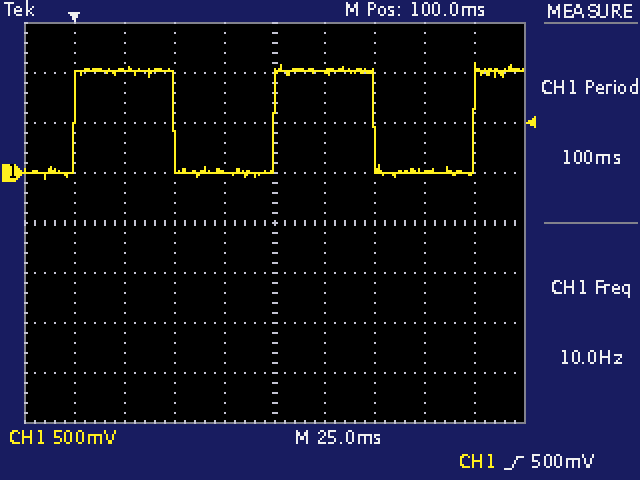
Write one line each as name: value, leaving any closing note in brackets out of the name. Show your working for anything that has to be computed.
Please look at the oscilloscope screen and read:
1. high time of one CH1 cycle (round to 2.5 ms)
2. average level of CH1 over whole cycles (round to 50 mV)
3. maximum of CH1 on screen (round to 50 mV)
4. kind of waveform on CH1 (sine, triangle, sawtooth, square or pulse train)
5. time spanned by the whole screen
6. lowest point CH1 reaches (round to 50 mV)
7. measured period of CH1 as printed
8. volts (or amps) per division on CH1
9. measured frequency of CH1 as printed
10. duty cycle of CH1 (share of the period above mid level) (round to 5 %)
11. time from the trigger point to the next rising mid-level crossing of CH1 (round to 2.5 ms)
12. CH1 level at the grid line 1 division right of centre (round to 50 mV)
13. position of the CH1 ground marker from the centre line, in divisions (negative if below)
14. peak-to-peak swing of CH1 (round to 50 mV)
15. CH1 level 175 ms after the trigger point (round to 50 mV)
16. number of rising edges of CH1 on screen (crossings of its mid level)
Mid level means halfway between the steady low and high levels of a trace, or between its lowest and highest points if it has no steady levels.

high time of one CH1 cycle: 50.0 ms
average level of CH1 over whole cycles: -50 mV + 0.5 × (1.10 V − (-50 mV)) ≈ 525 mV, so 500 mV to the nearest 50 mV
maximum of CH1 on screen: 1.10 V
kind of waveform on CH1: square
time spanned by the whole screen: 250 ms
lowest point CH1 reaches: -50 mV
measured period of CH1 as printed: 100 ms
volts (or amps) per division on CH1: 500 mV
measured frequency of CH1 as printed: 10.0 Hz
duty cycle of CH1 (share of the period above mid level): 50 %
time from the trigger point to the next rising mid-level crossing of CH1: 100.0 ms
CH1 level at the grid line 1 division right of centre: 1.00 V
position of the CH1 ground marker from the centre line, in divisions: +1.0 div
peak-to-peak swing of CH1: 1.10 V − (-50 mV) = 1.15 V
CH1 level 175 ms after the trigger point: 0 mV
number of rising edges of CH1 on screen: 3
